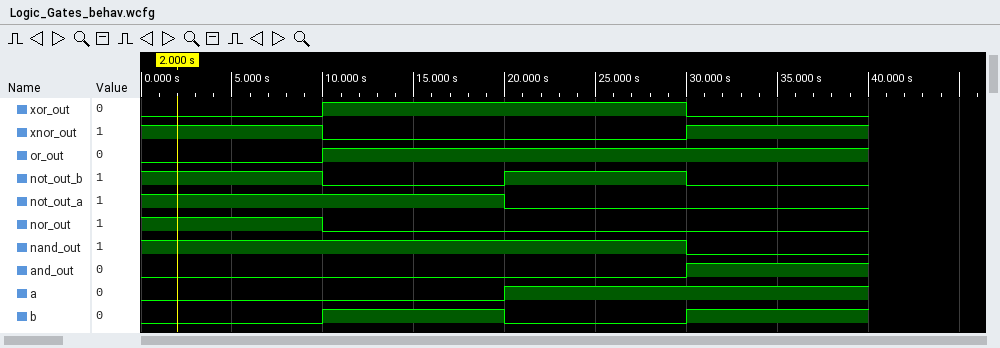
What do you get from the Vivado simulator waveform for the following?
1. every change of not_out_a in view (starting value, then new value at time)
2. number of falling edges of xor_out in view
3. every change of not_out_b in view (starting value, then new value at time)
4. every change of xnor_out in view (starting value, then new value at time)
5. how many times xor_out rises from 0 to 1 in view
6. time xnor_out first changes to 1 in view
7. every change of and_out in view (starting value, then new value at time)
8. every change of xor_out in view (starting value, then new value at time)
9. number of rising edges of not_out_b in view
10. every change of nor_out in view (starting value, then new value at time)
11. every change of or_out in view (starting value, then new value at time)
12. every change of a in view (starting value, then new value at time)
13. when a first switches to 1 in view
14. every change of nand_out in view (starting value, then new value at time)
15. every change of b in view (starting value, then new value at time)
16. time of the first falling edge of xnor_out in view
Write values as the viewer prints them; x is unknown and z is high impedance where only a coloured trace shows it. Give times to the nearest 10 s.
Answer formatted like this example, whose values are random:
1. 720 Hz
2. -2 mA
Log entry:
1. 1, 0 at 20 s
2. 1
3. 1, 0 at 10 s, 1 at 20 s, 0 at 30 s
4. 1, 0 at 10 s, 1 at 30 s
5. 1
6. 30 s
7. 0, 1 at 30 s
8. 0, 1 at 10 s, 0 at 30 s
9. 1
10. 1, 0 at 10 s
11. 0, 1 at 10 s
12. 0, 1 at 20 s
13. 20 s
14. 1, 0 at 30 s
15. 0, 1 at 10 s, 0 at 20 s, 1 at 30 s
16. 10 s
